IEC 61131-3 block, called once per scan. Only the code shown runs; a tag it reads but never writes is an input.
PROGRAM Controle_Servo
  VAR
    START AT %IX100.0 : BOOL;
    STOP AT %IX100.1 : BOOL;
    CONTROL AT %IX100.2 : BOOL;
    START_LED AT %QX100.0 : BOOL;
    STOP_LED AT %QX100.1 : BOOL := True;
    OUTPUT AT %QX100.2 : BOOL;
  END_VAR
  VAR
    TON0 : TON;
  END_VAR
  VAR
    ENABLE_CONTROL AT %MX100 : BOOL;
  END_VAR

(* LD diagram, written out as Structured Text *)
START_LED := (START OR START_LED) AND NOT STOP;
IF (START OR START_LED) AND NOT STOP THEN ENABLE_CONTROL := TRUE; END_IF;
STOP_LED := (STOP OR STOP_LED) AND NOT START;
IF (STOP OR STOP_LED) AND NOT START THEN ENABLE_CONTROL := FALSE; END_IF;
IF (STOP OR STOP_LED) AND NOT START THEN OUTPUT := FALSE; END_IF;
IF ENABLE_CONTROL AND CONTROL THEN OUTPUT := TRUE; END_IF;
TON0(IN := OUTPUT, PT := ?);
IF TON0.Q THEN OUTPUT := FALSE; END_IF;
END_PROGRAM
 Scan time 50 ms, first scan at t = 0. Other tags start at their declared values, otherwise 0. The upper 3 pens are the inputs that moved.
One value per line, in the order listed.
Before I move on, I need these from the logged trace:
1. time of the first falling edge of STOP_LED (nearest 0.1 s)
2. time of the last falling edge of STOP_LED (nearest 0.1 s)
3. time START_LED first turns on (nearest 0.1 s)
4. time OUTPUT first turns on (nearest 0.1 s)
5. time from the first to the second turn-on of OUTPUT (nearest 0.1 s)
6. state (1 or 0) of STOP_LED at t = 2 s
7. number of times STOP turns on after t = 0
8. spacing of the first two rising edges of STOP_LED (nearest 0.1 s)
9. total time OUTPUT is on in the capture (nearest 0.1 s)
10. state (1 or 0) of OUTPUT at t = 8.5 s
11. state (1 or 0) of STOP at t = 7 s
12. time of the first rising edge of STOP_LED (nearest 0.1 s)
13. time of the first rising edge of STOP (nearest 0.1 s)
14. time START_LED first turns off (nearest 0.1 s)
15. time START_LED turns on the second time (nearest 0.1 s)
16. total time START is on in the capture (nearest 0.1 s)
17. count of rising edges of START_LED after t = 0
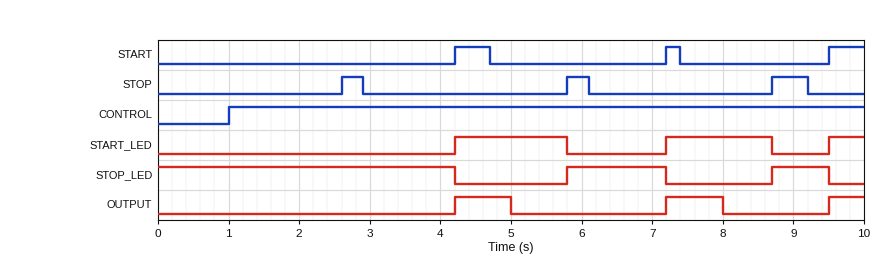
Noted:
4.2 s
9.5 s
4.2 s
4.2 s
3.0 s
1
3
2.9 s
2.1 s
0
0
5.8 s
2.6 s
5.8 s
7.2 s
1.2 s
3
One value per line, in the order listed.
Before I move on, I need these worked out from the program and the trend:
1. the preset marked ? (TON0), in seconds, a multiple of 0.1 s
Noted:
0.8 s
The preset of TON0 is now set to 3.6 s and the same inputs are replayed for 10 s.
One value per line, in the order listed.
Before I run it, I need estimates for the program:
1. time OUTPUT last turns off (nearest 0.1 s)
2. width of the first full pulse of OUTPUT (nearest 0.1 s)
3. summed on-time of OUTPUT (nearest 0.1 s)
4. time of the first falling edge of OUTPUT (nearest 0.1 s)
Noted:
8.7 s
1.6 s
3.6 s
5.8 s
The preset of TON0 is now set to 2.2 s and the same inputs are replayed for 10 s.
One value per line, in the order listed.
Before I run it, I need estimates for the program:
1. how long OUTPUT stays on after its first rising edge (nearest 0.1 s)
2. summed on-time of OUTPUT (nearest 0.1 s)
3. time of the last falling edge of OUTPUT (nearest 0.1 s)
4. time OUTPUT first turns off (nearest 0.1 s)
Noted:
1.6 s
3.6 s
8.7 s
5.8 s
